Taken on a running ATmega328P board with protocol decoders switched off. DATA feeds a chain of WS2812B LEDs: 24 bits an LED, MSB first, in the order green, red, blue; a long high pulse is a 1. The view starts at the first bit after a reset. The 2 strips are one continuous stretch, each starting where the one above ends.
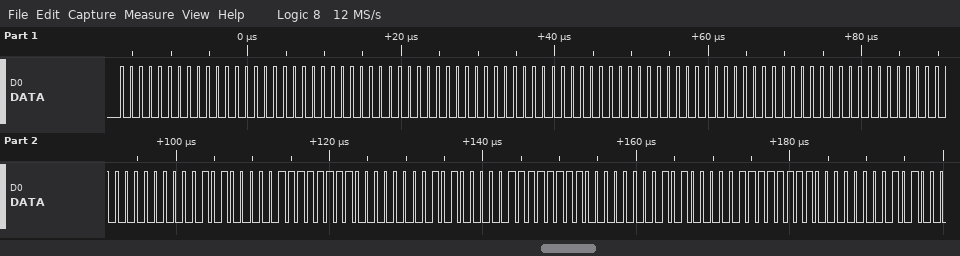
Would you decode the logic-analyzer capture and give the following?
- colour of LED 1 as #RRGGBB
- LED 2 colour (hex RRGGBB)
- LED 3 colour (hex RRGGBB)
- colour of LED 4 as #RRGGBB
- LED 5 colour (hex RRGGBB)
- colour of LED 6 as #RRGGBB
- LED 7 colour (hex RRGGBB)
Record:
#000000
#000000
#000000
#000000
#FFA000
#FFA000
#FFA000
